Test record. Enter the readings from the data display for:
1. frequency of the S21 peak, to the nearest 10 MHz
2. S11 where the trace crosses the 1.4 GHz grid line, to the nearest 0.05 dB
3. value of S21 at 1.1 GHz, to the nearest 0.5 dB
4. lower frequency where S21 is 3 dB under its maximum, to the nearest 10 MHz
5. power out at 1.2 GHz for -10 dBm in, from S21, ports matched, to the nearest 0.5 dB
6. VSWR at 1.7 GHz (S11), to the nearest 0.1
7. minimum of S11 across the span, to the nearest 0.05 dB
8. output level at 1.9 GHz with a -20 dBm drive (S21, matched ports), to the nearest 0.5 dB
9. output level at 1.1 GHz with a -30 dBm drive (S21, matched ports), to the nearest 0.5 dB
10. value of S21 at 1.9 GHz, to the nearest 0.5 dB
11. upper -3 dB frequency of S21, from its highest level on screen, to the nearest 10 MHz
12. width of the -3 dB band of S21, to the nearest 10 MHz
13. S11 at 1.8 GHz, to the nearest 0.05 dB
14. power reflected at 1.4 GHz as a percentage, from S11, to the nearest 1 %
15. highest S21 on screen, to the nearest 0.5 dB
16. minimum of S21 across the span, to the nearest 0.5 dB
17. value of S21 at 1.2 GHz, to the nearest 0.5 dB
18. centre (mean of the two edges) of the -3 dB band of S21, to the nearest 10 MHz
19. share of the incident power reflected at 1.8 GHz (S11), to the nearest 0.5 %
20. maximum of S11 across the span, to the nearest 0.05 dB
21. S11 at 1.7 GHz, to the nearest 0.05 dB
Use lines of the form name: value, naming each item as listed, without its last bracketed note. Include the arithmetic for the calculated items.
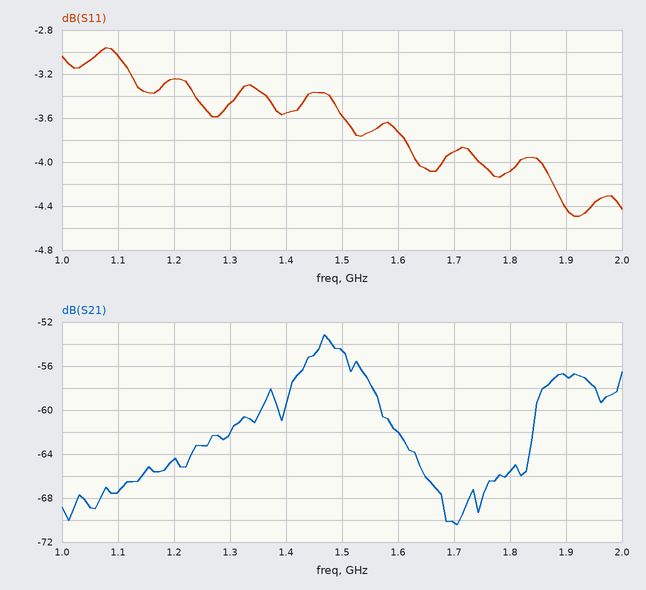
frequency of the S21 peak, to the nearest 10 MHz: 1.47 GHz
S11 where the trace crosses the 1.4 GHz grid line, to the nearest 0.05 dB: -3.55 dB
value of S21 at 1.1 GHz, to the nearest 0.5 dB: -67.5 dB
lower frequency where S21 is 3 dB under its maximum, to the nearest 10 MHz: 1.43 GHz
power out at 1.2 GHz for -10 dBm in, from S21, ports matched, to the nearest 0.5 dB: -10 dBm + (-64.5 dB) = -74.5 dBm
VSWR at 1.7 GHz (S11), to the nearest 0.1: |Γ| = 10^(-3.9/20) = 0.6383; VSWR = (1 + 0.6383)/(1 − 0.6383) ≈ 4.5
minimum of S11 across the span, to the nearest 0.05 dB: -4.50 dB
output level at 1.9 GHz with a -20 dBm drive (S21, matched ports), to the nearest 0.5 dB: -20 dBm + (-57.0 dB) = -77.0 dBm
output level at 1.1 GHz with a -30 dBm drive (S21, matched ports), to the nearest 0.5 dB: -30 dBm + (-67.5 dB) = -97.5 dBm
value of S21 at 1.9 GHz, to the nearest 0.5 dB: -57.0 dB
upper -3 dB frequency of S21, from its highest level on screen, to the nearest 10 MHz: 1.51 GHz
width of the -3 dB band of S21, to the nearest 10 MHz: 1.51 GHz − 1.43 GHz = 80 MHz
S11 at 1.8 GHz, to the nearest 0.05 dB: -4.10 dB
power reflected at 1.4 GHz as a percentage, from S11, to the nearest 1 %: 10^(-3.55/10) ≈ 44 %
highest S21 on screen, to the nearest 0.5 dB: -53.0 dB
minimum of S21 across the span, to the nearest 0.5 dB: -70.5 dB
value of S21 at 1.2 GHz, to the nearest 0.5 dB: -64.5 dB
centre (mean of the two edges) of the -3 dB band of S21, to the nearest 10 MHz: 1.47 GHz
share of the incident power reflected at 1.8 GHz (S11), to the nearest 0.5 %: 10^(-4.1/10) ≈ 38.9 %, so 39.0 % to the nearest 0.5 %
maximum of S11 across the span, to the nearest 0.05 dB: -2.95 dB
S11 at 1.7 GHz, to the nearest 0.05 dB: -3.90 dB
